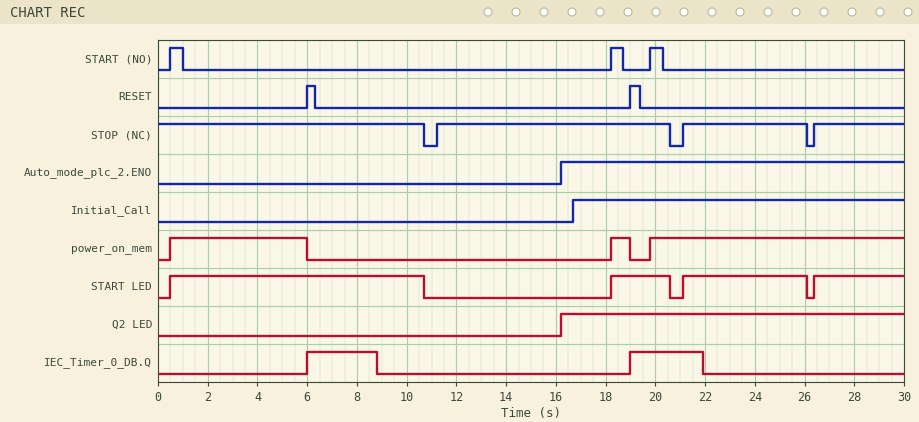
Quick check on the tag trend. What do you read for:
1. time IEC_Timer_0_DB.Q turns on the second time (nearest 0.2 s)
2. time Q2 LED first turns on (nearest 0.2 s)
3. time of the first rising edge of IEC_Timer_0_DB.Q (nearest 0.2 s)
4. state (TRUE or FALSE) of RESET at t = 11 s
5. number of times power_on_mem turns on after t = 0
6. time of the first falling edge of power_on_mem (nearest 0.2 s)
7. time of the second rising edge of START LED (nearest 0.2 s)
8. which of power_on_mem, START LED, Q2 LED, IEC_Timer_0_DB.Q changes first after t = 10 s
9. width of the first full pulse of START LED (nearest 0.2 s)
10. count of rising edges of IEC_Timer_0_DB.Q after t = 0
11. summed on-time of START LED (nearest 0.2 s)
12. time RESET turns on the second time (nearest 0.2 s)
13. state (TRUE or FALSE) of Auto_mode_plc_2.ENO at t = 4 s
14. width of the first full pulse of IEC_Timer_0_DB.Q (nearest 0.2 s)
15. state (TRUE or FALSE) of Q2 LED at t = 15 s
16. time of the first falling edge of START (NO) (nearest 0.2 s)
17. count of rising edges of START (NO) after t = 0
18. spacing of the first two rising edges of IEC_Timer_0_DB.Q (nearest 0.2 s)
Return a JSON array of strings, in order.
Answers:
["19.0 s", "16.2 s", "6.0 s", "FALSE", "3", "6.0 s", "18.2 s", "START LED", "10.2 s", "2", "21.2 s", "19.0 s", "FALSE", "2.8 s", "FALSE", "1.0 s", "3", "13.0 s"]
